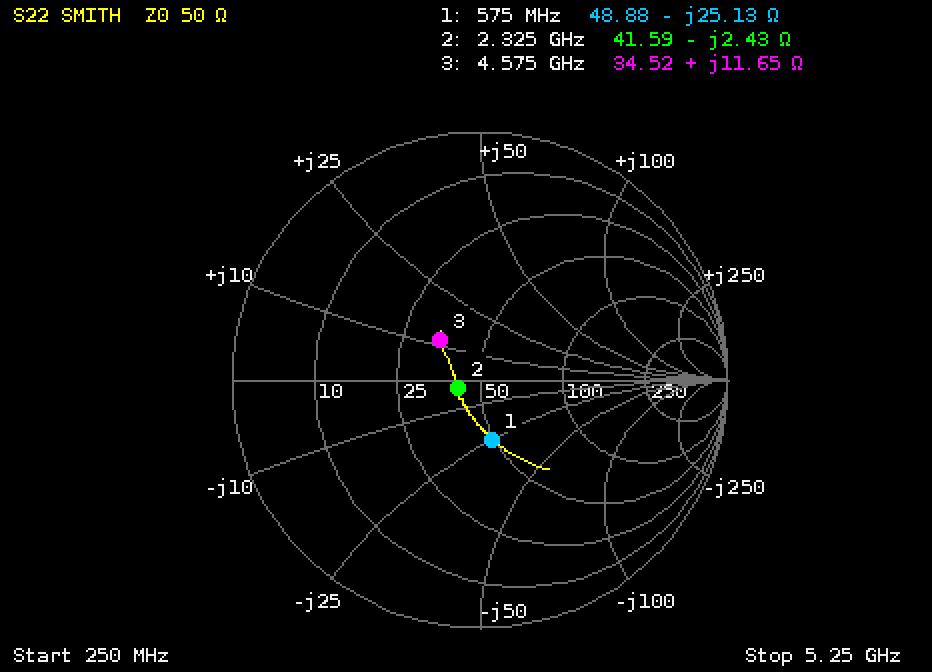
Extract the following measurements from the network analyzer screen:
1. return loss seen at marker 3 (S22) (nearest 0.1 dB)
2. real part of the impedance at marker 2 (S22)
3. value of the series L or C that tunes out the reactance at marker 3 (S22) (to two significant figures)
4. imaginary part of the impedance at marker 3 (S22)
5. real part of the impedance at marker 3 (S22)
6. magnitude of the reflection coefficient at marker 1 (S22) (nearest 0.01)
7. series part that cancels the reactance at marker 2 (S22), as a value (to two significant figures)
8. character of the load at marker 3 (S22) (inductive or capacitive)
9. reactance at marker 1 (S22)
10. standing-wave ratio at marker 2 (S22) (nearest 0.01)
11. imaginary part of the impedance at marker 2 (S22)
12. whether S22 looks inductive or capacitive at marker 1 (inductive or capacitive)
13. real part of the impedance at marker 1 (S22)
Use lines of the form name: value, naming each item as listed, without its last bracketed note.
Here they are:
return loss seen at marker 3 (S22): 12.9 dB
real part of the impedance at marker 2: 41.59 Ω
value of the series L or C that tunes out the reactance at marker 3 (S22): 3.0 pF
imaginary part of the impedance at marker 3: +11.65 Ω
real part of the impedance at marker 3: 34.52 Ω
magnitude of the reflection coefficient at marker 1 (S22): 0.25
series part that cancels the reactance at marker 2 (S22), as a value: 170 pH
character of the load at marker 3 (S22): inductive
reactance at marker 1: -25.13 Ω
standing-wave ratio at marker 2 (S22): 1.21
imaginary part of the impedance at marker 2: -2.43 Ω
whether S22 looks inductive or capacitive at marker 1: capacitive
real part of the impedance at marker 1: 48.88 Ω
